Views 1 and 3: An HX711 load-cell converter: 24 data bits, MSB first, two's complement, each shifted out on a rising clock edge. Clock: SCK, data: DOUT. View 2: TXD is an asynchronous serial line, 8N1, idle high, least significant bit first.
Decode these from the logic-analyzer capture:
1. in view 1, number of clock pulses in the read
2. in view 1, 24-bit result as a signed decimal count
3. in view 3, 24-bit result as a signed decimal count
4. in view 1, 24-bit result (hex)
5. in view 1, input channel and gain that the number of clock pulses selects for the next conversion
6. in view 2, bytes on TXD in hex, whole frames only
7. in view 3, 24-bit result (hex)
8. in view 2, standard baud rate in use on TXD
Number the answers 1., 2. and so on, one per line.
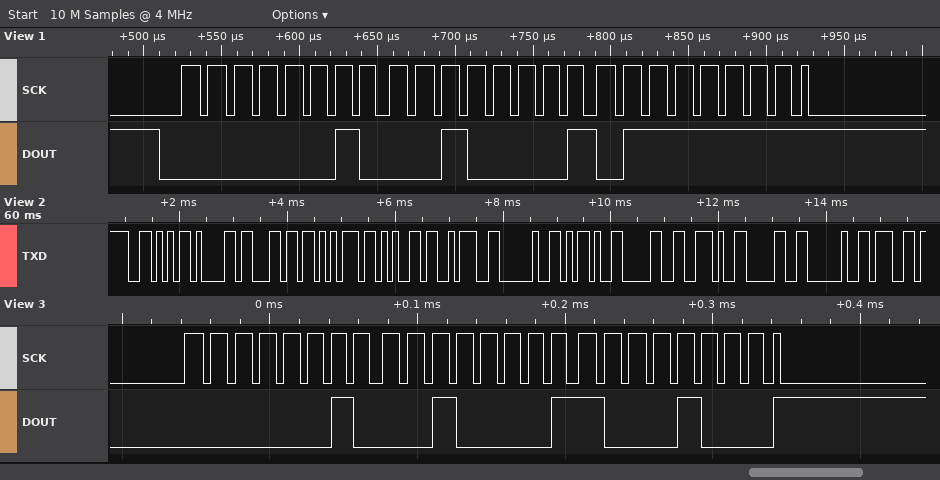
1. 25
2. 139647
3. 139656
4. 0x02217F
5. channel A, gain 128
6. 0x56 0x61 0x6C 0x75 0x65 0x3A 0x20 0x2D 0x30 0x2E 0x30 0x20 0x67
7. 0x022188
8. 9600 baud
